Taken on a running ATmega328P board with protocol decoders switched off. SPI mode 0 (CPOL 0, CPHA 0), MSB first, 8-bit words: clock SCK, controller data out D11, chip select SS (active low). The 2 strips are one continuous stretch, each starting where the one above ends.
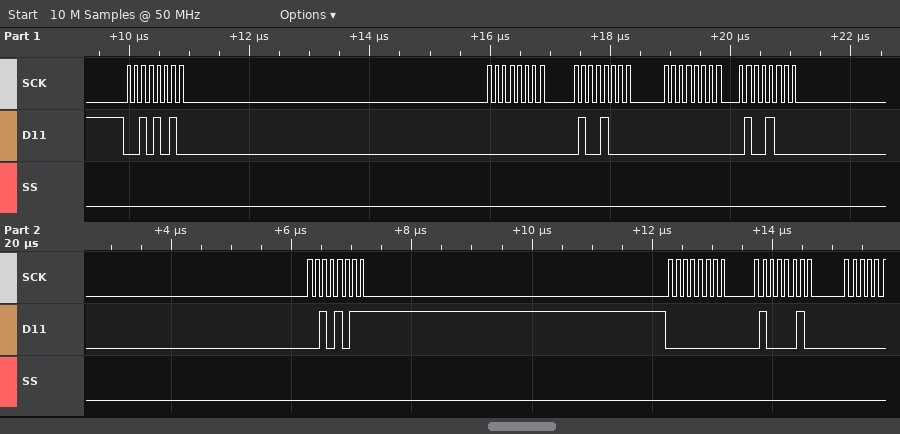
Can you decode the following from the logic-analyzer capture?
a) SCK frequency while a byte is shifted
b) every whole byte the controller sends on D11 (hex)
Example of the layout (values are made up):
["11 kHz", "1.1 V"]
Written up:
["8 MHz", "0x2A 0x00 0x48 0x00 0x48 0x2B 0x00 0x42"]
